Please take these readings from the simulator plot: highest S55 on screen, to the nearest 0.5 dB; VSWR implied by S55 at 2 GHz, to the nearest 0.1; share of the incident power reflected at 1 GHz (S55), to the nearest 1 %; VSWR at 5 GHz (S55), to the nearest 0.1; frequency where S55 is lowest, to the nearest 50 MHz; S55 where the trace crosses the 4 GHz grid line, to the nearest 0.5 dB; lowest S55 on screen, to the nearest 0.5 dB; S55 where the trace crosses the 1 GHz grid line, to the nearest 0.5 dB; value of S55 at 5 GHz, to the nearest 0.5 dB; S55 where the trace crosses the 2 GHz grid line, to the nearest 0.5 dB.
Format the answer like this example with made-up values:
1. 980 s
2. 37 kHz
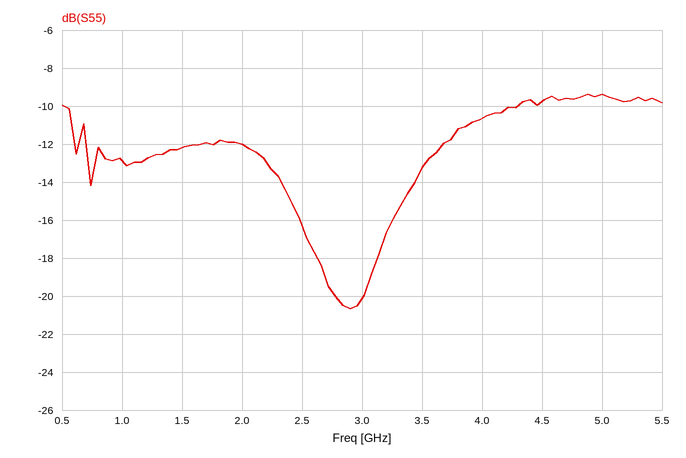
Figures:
1. -9.5 dB
2. 1.7
3. 5 %
4. 2.0
5. 2.90 GHz
6. -10.5 dB
7. -20.5 dB
8. -13.0 dB
9. -9.5 dB
10. -12.0 dB
